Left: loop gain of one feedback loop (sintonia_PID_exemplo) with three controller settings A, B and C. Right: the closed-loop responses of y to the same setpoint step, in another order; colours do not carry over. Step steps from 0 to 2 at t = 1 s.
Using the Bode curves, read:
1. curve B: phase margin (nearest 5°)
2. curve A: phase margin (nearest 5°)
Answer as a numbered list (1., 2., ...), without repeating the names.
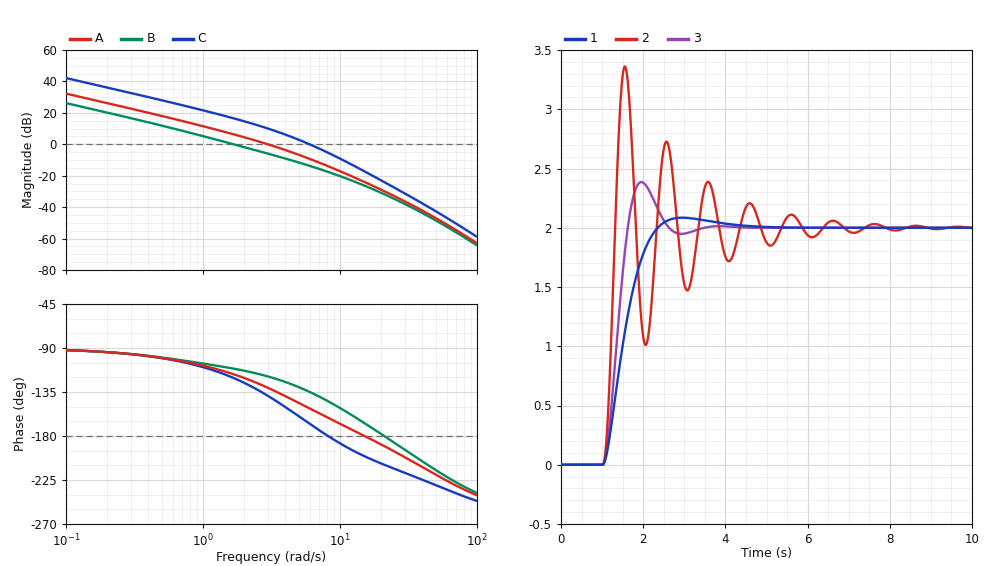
1. 70°
2. 50°
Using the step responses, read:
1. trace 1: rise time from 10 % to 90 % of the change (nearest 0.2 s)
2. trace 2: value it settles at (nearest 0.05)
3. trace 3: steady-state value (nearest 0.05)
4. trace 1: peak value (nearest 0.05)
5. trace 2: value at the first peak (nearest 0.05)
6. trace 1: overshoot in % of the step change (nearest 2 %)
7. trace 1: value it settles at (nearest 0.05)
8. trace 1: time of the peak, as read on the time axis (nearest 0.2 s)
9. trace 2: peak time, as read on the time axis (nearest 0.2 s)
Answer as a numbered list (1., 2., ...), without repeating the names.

1. 0.8 s
2. 2.00
3. 2.00
4. 2.10
5. 3.35
6. 4 %
7. 2.00
8. 3.0 s
9. 1.6 s
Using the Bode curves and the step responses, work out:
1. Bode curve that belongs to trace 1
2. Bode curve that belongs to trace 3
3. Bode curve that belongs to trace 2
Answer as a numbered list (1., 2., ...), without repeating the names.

1. B
2. A
3. C
